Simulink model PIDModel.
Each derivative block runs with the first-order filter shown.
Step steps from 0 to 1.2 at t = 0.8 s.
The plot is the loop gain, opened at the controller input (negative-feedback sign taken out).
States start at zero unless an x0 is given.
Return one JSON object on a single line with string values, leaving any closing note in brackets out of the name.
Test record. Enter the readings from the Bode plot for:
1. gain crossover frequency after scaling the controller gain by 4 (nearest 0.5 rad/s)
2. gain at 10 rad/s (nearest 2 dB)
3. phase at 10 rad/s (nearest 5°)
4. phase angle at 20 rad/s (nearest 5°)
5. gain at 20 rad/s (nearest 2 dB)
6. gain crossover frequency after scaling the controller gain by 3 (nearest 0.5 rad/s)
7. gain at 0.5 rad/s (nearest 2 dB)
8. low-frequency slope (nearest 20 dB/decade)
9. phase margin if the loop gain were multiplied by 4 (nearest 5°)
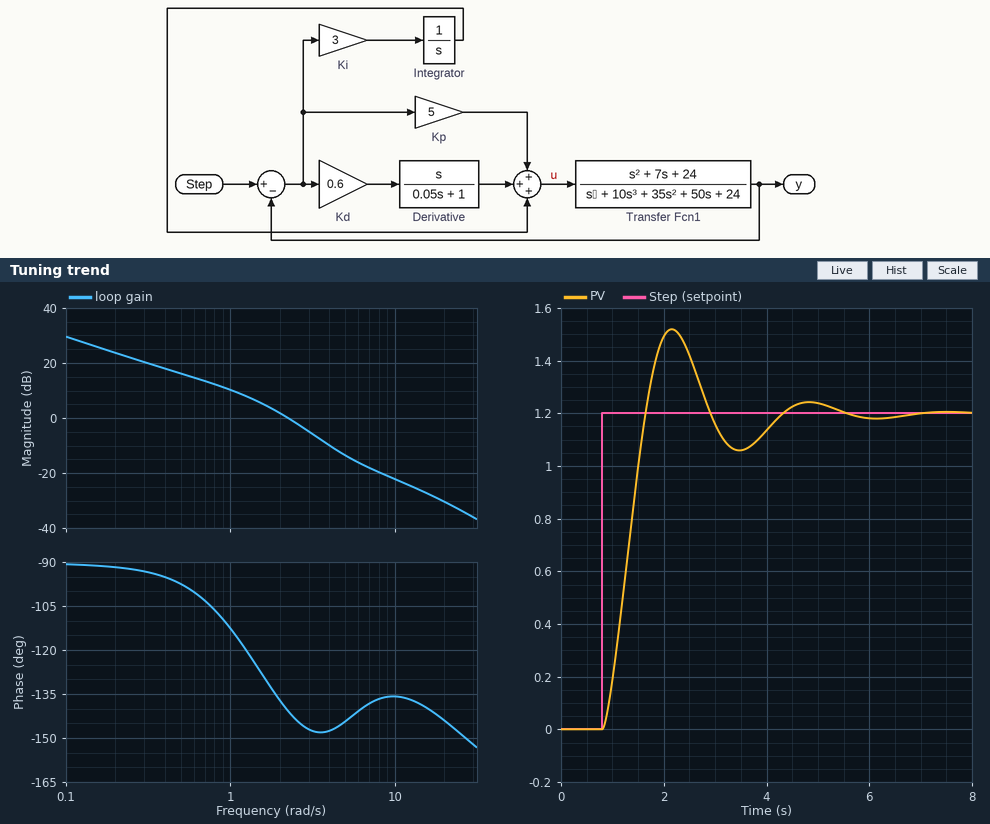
{"gain crossover frequency after scaling the controller gain by 4": "4.5 rad/s", "gain at 10 rad/s": "-22 dB", "phase at 10 rad/s": "-135°", "phase angle at 20 rad/s": "-145°", "gain at 20 rad/s": "-30 dB", "gain crossover frequency after scaling the controller gain by 3": "4.0 rad/s", "gain at 0.5 rad/s": "16 dB", "low-frequency slope": "-20 dB/decade", "phase margin if the loop gain were multiplied by 4": "35°"}
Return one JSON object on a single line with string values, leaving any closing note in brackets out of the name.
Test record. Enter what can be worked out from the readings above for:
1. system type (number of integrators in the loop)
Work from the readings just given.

{"system type": "1"}
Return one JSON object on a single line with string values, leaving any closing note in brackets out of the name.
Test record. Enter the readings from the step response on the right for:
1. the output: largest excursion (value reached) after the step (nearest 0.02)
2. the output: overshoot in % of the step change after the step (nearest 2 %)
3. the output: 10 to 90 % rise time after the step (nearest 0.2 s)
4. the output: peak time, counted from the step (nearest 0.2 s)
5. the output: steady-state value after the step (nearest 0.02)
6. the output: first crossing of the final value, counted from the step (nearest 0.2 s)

{"the output: largest excursion (value reached) after the step": "1.52", "the output: overshoot in % of the step change after the step": "26 %", "the output: 10 to 90 % rise time after the step": "0.6 s", "the output: peak time, counted from the step": "1.4 s", "the output: steady-state value after the step": "1.20", "the output: first crossing of the final value, counted from the step": "0.8 s"}
